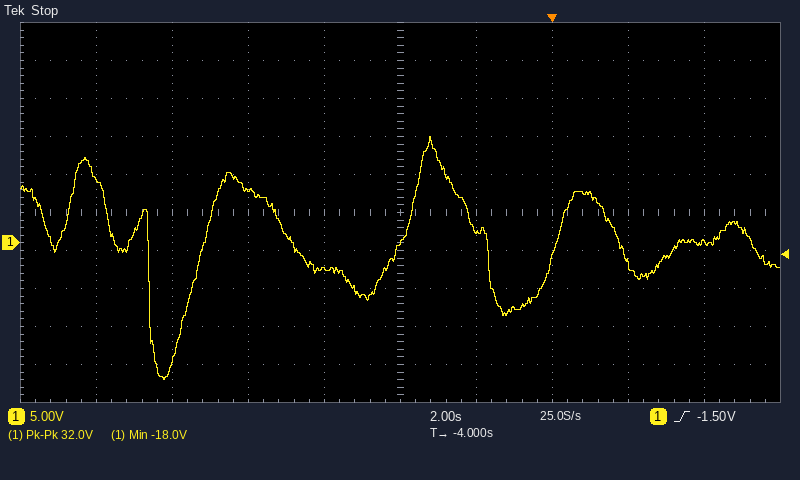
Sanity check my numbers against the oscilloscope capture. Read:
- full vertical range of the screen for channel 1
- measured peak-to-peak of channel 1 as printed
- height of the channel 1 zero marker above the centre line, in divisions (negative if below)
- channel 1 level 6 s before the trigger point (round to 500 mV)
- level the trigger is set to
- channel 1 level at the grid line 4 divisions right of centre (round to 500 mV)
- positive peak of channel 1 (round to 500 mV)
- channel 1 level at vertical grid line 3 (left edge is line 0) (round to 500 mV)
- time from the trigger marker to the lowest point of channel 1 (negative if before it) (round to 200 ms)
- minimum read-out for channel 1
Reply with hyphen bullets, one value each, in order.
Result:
- 50 V
- 32.0 V
- -0.8 div
- -3.5 V
- -1.50 V
- 0.0 V
- 14.0 V
- 7.0 V
- -10.2 s
- -18.0 V
